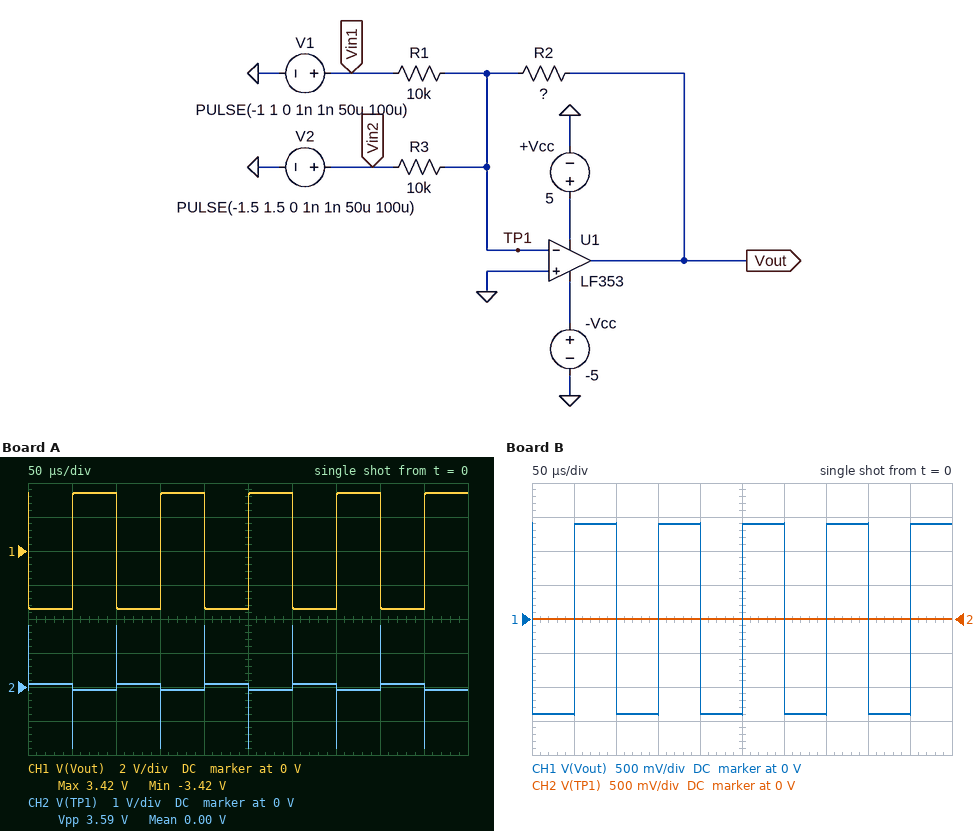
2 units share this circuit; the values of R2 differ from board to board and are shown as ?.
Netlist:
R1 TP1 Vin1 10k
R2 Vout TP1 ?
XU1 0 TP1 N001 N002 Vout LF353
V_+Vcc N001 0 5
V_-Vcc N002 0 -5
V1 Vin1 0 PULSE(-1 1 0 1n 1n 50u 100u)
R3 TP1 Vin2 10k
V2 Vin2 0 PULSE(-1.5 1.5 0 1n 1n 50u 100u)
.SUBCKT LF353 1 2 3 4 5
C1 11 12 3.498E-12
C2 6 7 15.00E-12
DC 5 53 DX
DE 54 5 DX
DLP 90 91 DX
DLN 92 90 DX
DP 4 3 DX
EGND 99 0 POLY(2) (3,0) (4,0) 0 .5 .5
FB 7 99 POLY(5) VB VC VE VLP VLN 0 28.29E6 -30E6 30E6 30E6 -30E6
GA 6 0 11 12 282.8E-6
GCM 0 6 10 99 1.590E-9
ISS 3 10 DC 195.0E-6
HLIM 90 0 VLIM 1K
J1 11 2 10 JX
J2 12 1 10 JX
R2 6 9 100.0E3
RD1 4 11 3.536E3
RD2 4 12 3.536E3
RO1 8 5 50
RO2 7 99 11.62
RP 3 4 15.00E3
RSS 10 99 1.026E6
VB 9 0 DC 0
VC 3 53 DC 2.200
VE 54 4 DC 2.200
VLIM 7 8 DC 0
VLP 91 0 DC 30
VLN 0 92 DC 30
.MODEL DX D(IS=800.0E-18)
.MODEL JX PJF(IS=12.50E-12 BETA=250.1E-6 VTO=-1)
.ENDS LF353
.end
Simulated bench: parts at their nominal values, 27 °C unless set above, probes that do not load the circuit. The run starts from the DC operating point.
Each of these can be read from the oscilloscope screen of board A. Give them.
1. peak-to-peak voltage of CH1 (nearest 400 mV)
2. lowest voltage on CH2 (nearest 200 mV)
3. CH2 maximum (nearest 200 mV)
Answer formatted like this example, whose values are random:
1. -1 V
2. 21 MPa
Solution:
1. 6.8 V
2. -1.8 V
3. 1.8 V
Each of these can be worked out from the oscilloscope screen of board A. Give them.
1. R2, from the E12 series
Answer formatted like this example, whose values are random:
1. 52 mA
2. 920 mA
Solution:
1. 15 kΩ
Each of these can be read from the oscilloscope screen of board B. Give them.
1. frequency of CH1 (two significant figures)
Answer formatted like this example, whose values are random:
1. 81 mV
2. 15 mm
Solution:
1. 10 kHz
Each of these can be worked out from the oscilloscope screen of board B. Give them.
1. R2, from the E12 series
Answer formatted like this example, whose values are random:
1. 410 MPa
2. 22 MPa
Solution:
1. 5.6 kΩ
